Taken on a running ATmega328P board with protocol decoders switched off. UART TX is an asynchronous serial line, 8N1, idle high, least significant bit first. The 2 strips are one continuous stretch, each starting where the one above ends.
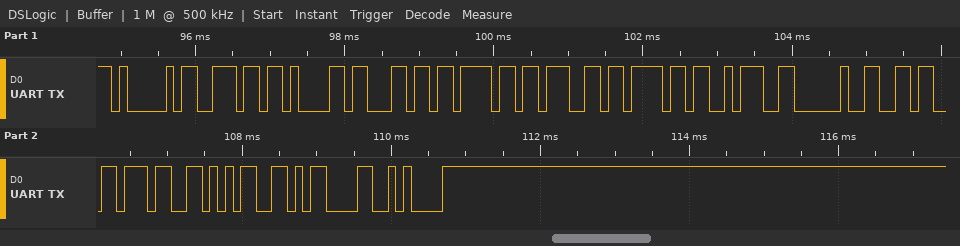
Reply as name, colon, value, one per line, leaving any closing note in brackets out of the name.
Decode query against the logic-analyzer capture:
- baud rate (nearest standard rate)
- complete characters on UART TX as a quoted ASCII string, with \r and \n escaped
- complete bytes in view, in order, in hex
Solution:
baud rate: 9600 baud
complete characters on UART TX as a quoted ASCII string, with \r and \n escaped: "Analogo: 675\r\n"
complete bytes in view, in order, in hex: 0x41 0x6E 0x61 0x6C 0x6F 0x67 0x6F 0x3A 0x20 0x36 0x37 0x35 0x0D 0x0A
